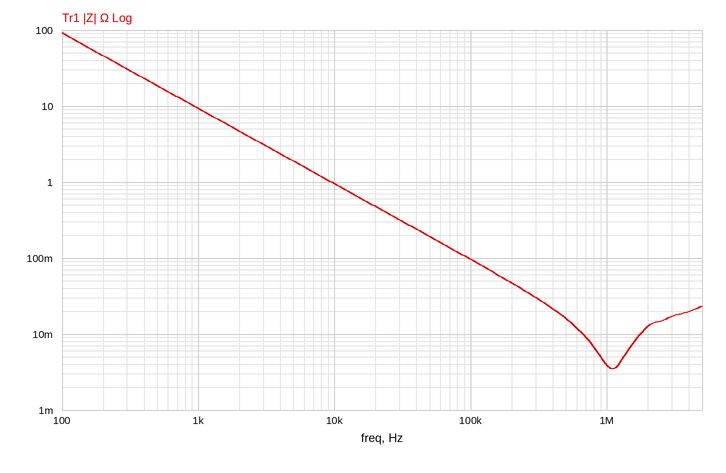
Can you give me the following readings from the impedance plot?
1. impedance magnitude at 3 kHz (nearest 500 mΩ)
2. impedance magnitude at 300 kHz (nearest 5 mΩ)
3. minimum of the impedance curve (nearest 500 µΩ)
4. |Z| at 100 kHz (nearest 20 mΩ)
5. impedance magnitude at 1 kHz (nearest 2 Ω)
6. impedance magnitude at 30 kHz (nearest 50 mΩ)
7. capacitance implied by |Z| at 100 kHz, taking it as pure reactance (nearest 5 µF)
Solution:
3.0 Ω
30 mΩ
3.5 mΩ
100 mΩ
10 Ω
300 mΩ
15 µF
